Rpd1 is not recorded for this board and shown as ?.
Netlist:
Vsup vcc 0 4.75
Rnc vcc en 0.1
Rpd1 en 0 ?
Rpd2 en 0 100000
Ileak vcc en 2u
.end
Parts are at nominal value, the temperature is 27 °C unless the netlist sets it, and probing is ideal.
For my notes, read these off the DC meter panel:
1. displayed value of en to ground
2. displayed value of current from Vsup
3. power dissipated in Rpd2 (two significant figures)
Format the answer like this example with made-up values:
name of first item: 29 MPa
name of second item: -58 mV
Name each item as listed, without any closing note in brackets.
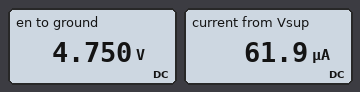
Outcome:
displayed value of en to ground: 4.750 V
displayed value of current from Vsup: 61.9 µA
power dissipated in Rpd2: 230 µW
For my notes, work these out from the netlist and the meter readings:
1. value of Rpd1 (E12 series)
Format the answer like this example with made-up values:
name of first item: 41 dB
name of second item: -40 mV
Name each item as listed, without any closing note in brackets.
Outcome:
value of Rpd1: 330 kΩ
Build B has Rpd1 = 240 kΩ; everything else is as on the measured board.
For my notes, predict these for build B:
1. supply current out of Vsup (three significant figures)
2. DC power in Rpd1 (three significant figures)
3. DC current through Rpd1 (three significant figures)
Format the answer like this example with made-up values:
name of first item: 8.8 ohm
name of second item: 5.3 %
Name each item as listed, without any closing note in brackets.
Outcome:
supply current out of Vsup: 67.3 µA
DC power in Rpd1: 94.0 µW
DC current through Rpd1: 19.8 µA
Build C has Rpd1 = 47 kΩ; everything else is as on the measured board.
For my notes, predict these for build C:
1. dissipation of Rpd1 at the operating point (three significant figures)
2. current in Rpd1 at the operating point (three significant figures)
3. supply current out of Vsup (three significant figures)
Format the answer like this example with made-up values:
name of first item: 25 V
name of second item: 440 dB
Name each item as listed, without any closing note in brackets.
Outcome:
dissipation of Rpd1 at the operating point: 480 µW
current in Rpd1 at the operating point: 101 µA
supply current out of Vsup: 149 µA
